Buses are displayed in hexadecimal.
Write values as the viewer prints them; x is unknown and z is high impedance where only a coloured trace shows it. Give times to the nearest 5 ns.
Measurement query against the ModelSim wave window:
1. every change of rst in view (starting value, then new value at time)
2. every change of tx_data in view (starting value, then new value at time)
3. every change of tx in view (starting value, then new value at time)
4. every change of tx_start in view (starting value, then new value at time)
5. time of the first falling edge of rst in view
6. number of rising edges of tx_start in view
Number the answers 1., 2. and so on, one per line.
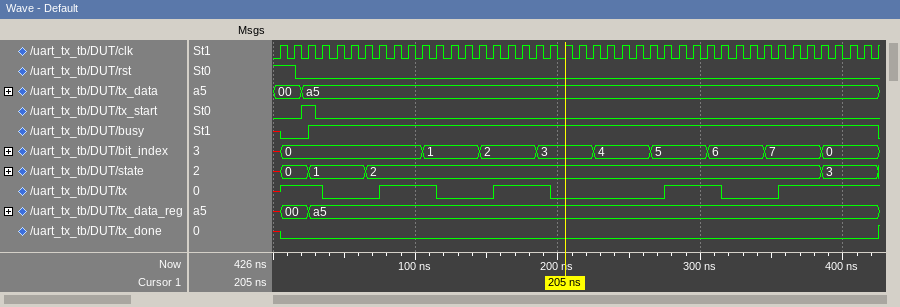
1. 1, 0 at 15 ns
2. 00, a5 at 20 ns
3. x, 1 at 5 ns, 0 at 35 ns, 1 at 75 ns, 0 at 115 ns, 1 at 155 ns, 0 at 195 ns, 1 at 275 ns, 0 at 315 ns, 1 at 355 ns
4. 0, 1 at 20 ns, 0 at 30 ns
5. 15 ns
6. 1
